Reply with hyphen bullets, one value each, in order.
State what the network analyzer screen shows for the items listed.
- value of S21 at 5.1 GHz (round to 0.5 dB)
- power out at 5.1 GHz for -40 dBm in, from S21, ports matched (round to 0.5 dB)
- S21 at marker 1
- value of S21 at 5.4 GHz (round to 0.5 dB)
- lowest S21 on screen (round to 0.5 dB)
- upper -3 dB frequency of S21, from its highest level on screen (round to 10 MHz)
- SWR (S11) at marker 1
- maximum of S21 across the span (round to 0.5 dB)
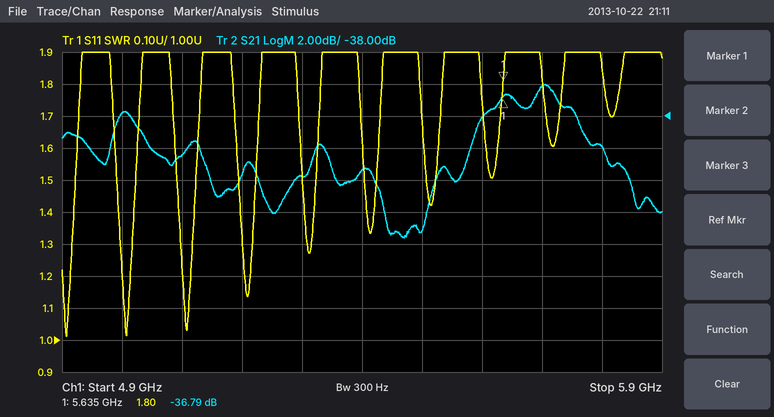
- -40.5 dB
- -80.5 dBm
- -36.79 dB
- -41.5 dB
- -45.5 dB
- 5.77 GHz
- 1.80
- -36.0 dB
